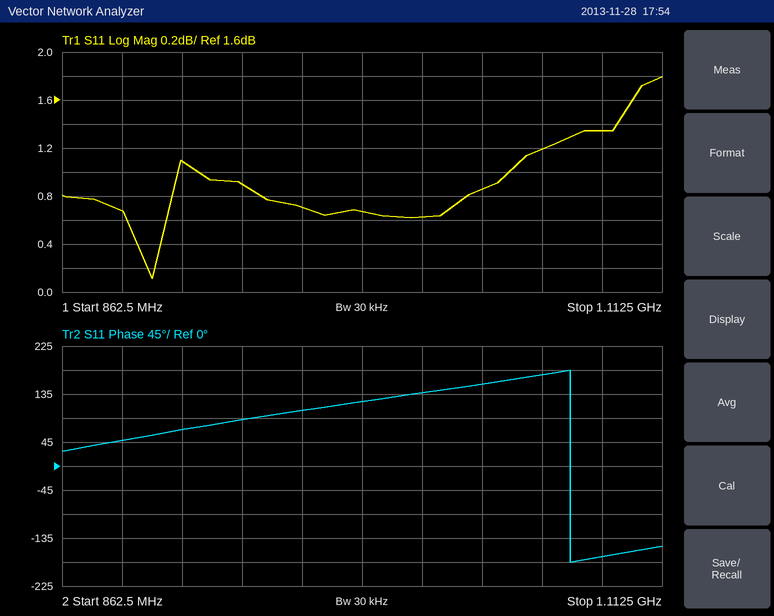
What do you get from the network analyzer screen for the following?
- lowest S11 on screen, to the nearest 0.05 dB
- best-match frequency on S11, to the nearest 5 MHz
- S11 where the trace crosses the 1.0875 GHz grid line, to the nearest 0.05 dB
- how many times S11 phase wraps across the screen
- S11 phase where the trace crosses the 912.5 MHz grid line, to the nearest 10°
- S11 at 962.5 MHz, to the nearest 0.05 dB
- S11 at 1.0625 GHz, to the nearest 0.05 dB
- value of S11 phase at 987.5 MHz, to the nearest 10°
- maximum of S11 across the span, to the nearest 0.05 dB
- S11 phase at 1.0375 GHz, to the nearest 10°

0.10 dB
900 MHz
1.35 dB
1
70°
0.70 dB
1.20 dB
120°
1.80 dB
150°
